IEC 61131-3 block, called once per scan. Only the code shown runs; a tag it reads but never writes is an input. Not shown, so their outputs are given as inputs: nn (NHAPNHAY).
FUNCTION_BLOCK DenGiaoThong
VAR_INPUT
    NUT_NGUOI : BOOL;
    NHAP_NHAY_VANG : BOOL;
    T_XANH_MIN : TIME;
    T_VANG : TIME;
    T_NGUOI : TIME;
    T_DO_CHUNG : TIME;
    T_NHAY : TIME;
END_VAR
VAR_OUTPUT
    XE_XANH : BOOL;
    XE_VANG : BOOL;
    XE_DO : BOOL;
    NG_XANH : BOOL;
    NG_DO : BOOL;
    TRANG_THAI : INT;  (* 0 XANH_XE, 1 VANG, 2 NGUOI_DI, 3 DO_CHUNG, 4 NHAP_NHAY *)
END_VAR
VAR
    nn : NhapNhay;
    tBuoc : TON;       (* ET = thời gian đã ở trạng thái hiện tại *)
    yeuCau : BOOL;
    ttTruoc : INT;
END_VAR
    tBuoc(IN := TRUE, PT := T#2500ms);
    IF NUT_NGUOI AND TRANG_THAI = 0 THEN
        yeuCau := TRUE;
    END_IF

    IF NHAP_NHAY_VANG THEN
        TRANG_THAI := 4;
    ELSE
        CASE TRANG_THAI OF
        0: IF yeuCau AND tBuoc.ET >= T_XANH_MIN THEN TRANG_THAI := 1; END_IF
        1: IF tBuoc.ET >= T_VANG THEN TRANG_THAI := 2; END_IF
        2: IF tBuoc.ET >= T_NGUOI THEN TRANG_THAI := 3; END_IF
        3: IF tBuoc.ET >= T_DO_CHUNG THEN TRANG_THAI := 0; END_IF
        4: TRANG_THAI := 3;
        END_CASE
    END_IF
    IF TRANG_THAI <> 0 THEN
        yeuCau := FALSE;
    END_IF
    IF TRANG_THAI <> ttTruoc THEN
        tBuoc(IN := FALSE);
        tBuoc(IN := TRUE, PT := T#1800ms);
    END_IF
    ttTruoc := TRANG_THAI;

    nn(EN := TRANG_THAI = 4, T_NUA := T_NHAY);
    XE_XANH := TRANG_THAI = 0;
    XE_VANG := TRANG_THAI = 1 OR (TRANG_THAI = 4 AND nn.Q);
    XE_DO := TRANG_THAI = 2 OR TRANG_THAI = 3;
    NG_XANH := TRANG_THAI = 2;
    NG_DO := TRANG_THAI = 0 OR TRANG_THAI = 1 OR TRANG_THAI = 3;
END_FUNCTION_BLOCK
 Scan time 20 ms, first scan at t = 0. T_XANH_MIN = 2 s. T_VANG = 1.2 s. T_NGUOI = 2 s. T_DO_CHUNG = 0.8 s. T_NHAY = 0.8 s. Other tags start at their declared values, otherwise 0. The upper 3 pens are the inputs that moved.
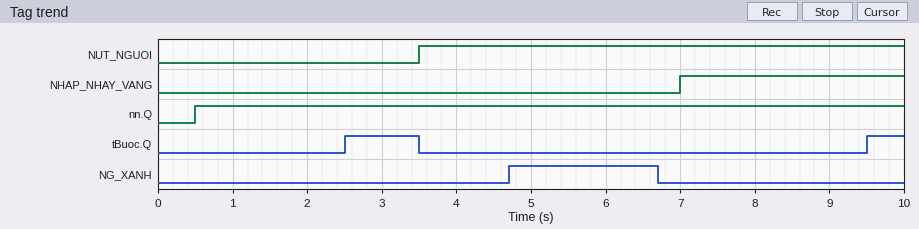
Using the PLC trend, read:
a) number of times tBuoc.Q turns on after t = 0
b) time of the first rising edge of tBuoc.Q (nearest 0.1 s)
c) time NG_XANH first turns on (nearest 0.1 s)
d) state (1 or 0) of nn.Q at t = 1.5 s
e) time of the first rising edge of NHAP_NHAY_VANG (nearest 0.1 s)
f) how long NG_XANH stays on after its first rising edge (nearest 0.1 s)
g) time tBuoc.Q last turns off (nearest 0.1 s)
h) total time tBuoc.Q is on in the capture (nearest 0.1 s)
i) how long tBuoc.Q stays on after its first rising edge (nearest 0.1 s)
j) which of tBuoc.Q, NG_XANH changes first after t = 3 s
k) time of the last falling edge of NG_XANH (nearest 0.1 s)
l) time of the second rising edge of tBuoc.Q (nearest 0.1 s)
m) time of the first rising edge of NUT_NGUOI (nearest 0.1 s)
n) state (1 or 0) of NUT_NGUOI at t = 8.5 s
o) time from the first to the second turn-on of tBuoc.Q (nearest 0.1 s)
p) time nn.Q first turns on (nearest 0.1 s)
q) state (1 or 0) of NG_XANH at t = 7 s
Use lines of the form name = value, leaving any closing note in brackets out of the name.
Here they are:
number of times tBuoc.Q turns on after t = 0 = 2
time of the first rising edge of tBuoc.Q = 2.5 s
time NG_XANH first turns on = 4.7 s
state (1 or 0) of nn.Q at t = 1.5 s = 1
time of the first rising edge of NHAP_NHAY_VANG = 7.0 s
how long NG_XANH stays on after its first rising edge = 2.0 s
time tBuoc.Q last turns off = 3.5 s
total time tBuoc.Q is on in the capture = 1.5 s
how long tBuoc.Q stays on after its first rising edge = 1.0 s
which of tBuoc.Q, NG_XANH changes first after t = 3 s = tBuoc.Q
time of the last falling edge of NG_XANH = 6.7 s
time of the second rising edge of tBuoc.Q = 9.5 s
time of the first rising edge of NUT_NGUOI = 3.5 s
state (1 or 0) of NUT_NGUOI at t = 8.5 s = 1
time from the first to the second turn-on of tBuoc.Q = 7.0 s
time nn.Q first turns on = 0.5 s
state (1 or 0) of NG_XANH at t = 7 s = 0
